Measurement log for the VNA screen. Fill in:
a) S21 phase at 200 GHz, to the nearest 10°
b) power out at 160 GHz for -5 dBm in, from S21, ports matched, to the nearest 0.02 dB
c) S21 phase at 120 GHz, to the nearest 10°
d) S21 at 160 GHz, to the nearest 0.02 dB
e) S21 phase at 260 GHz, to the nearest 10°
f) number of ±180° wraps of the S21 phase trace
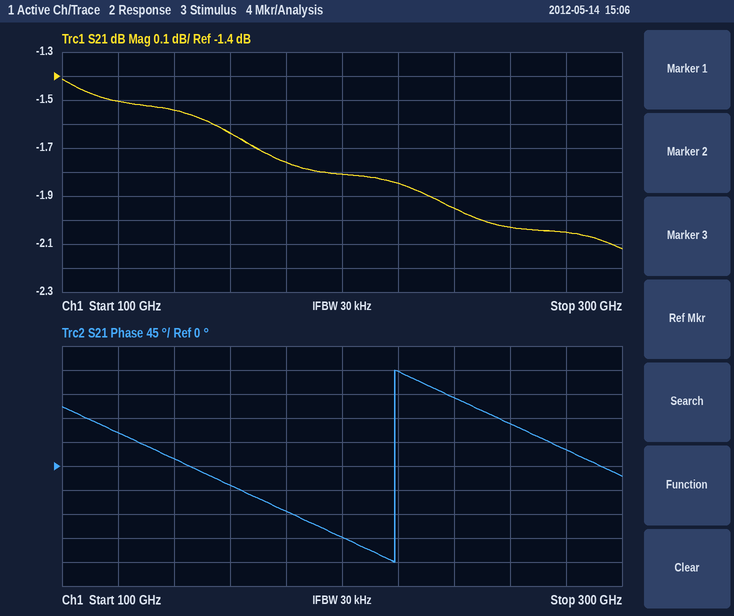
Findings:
-130°
-6.64 dBm
60°
-1.64 dB
80°
1
